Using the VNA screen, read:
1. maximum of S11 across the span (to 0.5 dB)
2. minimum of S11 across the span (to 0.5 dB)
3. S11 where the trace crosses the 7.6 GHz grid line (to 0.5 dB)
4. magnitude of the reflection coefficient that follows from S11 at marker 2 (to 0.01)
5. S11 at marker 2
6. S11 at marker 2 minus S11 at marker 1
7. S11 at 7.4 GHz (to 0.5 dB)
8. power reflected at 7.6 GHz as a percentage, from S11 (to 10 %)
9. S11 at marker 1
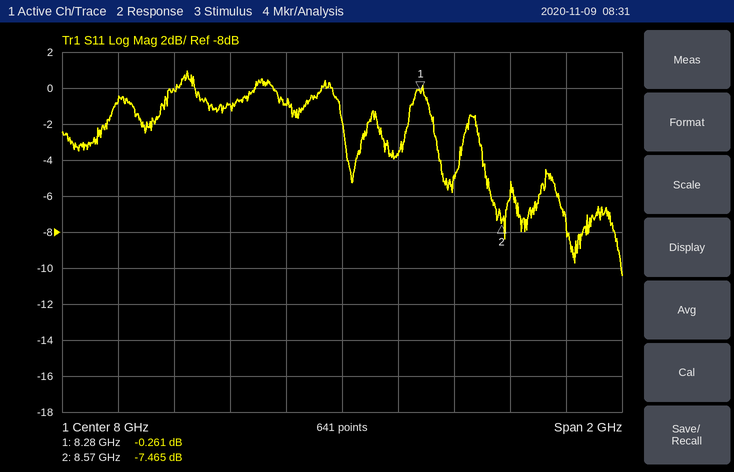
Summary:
1.0 dB
-10.5 dB
-1.0 dB
0.42
-7.465 dB
-7.204 dB
0.0 dB
80 %
-0.261 dB
